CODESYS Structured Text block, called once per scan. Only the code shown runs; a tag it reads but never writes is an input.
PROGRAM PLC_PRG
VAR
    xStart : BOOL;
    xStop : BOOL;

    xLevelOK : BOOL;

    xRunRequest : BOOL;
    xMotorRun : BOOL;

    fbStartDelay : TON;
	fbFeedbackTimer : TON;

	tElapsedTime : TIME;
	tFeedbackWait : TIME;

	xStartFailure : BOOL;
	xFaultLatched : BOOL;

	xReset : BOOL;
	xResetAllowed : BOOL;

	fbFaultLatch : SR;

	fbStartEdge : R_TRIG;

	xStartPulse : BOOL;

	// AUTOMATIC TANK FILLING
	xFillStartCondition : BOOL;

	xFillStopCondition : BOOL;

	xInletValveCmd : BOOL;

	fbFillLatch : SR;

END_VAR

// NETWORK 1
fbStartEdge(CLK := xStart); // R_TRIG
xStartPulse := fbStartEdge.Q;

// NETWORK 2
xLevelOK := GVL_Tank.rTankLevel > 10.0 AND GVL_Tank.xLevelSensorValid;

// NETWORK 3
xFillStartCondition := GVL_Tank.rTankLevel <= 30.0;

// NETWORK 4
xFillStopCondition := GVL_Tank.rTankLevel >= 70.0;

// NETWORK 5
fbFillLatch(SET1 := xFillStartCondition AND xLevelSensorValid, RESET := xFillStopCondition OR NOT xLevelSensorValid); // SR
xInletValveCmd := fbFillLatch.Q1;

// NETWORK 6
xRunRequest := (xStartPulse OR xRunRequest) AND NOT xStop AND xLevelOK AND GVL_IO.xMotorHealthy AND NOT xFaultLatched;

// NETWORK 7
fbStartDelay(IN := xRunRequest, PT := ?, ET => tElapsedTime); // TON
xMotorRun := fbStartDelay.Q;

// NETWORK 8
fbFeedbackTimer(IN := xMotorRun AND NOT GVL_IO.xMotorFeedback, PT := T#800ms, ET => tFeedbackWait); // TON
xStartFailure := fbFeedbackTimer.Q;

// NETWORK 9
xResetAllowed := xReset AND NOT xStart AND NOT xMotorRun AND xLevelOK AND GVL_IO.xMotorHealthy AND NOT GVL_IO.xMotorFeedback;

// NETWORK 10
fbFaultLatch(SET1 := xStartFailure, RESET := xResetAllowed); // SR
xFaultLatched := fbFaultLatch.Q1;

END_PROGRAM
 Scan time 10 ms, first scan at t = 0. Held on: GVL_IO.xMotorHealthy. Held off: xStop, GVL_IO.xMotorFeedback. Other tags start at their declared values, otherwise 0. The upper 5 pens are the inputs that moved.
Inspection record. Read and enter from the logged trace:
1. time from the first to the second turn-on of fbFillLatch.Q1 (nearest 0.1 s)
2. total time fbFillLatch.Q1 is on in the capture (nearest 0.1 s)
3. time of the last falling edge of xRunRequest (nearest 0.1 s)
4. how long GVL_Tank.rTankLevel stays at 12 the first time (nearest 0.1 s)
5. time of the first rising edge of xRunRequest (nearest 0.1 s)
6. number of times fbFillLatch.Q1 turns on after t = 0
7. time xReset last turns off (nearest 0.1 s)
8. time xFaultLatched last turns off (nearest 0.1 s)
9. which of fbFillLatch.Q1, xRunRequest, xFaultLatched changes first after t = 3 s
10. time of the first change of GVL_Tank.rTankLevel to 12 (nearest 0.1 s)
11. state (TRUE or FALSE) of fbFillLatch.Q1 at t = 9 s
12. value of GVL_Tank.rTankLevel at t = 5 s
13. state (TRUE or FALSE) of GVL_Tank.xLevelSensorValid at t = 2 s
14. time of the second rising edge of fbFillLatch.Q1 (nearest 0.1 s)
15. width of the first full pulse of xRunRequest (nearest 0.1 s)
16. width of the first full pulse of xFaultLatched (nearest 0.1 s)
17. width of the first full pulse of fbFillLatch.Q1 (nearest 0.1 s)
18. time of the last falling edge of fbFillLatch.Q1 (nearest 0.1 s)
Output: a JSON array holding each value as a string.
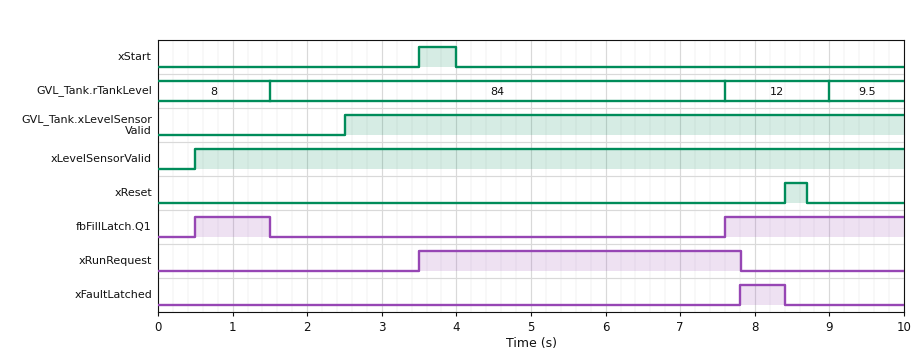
["7.1 s", "3.4 s", "7.8 s", "1.4 s", "3.5 s", "2", "8.7 s", "8.4 s", "xRunRequest", "7.6 s", "TRUE", "84", "FALSE", "7.6 s", "4.3 s", "0.6 s", "1.0 s", "1.5 s"]
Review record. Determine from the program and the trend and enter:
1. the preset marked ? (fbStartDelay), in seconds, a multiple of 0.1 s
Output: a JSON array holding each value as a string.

["3.5 s"]
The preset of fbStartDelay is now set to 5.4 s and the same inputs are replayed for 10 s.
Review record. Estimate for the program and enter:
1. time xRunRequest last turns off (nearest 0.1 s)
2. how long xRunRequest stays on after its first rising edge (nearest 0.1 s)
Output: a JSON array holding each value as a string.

["9.0 s", "5.5 s"]
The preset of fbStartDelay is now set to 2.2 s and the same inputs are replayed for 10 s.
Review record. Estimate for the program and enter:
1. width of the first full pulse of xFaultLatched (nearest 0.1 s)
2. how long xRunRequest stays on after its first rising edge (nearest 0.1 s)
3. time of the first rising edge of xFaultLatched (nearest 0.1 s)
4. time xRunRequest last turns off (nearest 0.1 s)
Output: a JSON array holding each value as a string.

["1.9 s", "3.0 s", "6.5 s", "6.5 s"]
